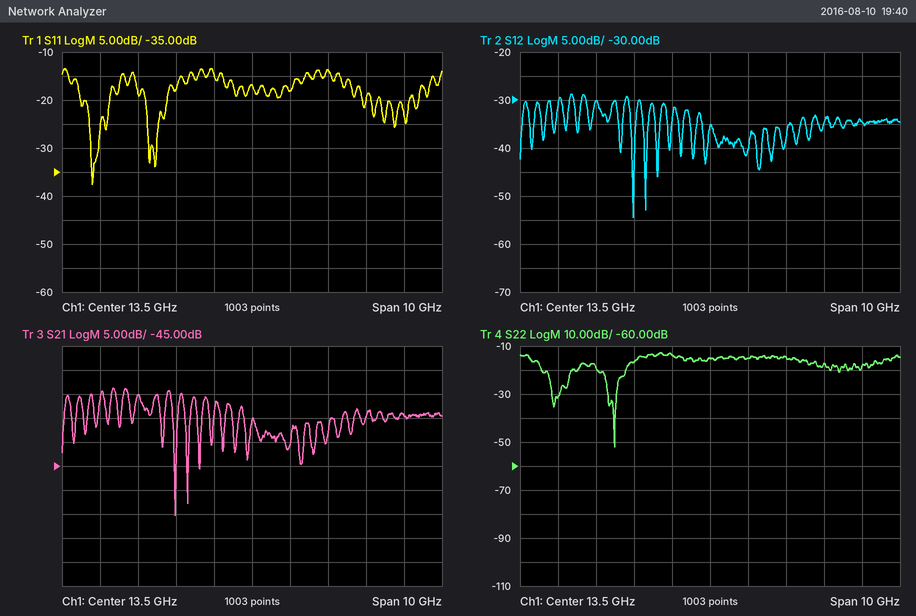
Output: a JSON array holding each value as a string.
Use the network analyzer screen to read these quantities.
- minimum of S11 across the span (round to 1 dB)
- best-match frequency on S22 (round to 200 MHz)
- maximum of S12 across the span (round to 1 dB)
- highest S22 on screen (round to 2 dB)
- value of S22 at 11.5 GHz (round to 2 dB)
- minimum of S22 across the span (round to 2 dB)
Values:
["-38 dB", "11.0 GHz", "-29 dB", "-12 dB", "-16 dB", "-52 dB"]
